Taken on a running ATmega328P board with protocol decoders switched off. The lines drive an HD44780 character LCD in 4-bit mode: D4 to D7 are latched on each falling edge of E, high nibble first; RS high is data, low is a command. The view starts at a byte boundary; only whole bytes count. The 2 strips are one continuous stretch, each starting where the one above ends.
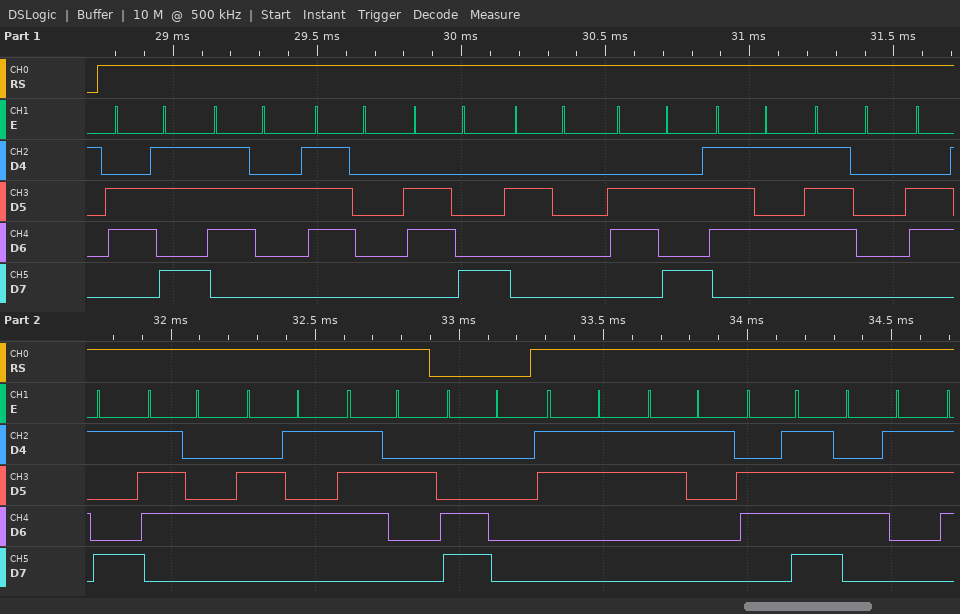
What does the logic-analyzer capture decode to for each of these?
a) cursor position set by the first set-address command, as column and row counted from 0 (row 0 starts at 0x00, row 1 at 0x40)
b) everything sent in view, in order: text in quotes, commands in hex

column 0, row 1
"krph jupiter" 0xC0 "31oc"
